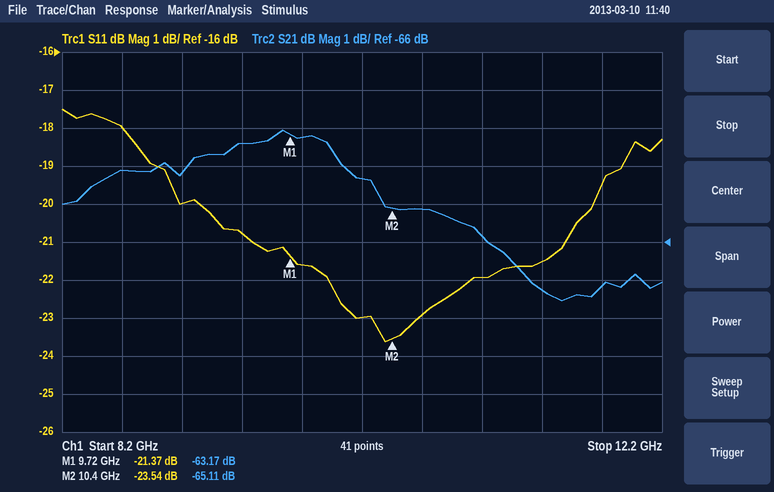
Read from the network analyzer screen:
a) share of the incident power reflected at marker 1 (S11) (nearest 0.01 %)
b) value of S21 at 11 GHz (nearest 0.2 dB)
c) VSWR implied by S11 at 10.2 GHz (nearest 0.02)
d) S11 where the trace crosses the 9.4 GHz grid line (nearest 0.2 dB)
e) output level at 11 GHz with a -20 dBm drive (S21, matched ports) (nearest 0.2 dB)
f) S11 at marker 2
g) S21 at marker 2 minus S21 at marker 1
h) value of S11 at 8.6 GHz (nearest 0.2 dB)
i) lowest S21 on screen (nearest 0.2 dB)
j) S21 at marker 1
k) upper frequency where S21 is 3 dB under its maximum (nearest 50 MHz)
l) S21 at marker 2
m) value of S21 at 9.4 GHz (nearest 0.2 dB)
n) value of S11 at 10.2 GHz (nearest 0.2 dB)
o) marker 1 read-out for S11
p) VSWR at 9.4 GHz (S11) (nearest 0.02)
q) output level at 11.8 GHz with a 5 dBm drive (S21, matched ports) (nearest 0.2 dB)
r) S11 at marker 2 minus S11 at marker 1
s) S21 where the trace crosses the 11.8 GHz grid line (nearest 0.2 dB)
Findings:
0.73 %
-65.8 dB
1.16
-20.8 dB
-85.8 dBm
-23.54 dB
-1.94 dB
-18.0 dB
-67.6 dB
-63.17 dB
11.05 GHz
-65.11 dB
-63.4 dB
-23.0 dB
-21.37 dB
1.20
-62.2 dBm
-2.17 dB
-67.2 dB
